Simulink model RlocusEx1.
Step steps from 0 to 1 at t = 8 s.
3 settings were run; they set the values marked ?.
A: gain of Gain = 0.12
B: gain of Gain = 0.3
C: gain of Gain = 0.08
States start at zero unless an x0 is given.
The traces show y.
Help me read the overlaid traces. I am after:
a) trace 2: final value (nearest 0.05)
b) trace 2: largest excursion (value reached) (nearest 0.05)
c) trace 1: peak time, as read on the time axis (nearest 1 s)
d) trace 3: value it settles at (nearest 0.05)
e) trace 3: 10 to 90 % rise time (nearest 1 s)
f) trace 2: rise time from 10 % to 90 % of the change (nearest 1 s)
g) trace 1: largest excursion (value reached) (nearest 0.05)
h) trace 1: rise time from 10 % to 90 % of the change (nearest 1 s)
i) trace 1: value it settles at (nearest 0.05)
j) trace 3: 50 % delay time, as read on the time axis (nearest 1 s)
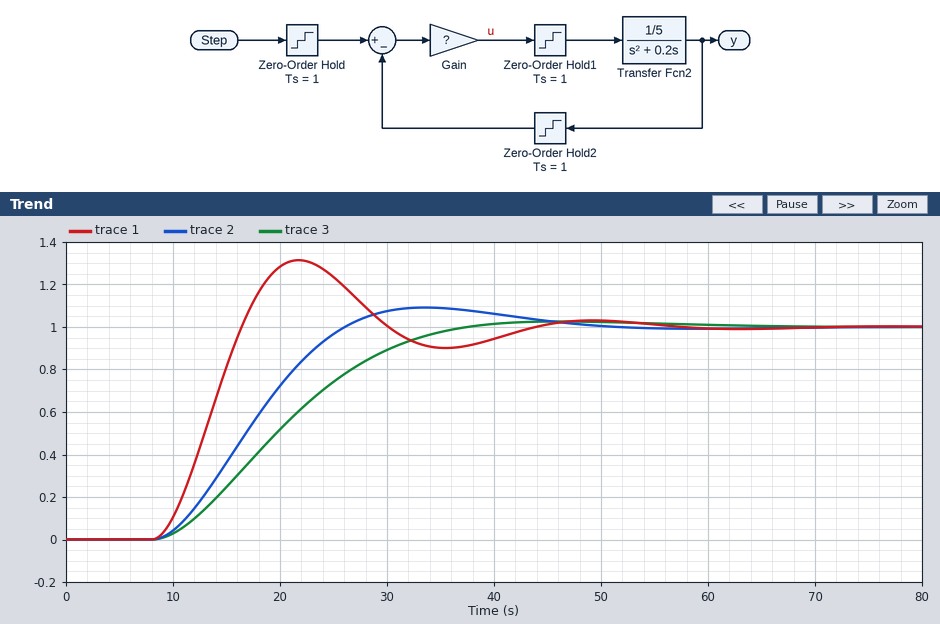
1.00
1.10
22 s
1.00
18 s
12 s
1.30
6 s
1.00
20 s
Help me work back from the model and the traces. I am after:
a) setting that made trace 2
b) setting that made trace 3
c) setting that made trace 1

A
C
B
